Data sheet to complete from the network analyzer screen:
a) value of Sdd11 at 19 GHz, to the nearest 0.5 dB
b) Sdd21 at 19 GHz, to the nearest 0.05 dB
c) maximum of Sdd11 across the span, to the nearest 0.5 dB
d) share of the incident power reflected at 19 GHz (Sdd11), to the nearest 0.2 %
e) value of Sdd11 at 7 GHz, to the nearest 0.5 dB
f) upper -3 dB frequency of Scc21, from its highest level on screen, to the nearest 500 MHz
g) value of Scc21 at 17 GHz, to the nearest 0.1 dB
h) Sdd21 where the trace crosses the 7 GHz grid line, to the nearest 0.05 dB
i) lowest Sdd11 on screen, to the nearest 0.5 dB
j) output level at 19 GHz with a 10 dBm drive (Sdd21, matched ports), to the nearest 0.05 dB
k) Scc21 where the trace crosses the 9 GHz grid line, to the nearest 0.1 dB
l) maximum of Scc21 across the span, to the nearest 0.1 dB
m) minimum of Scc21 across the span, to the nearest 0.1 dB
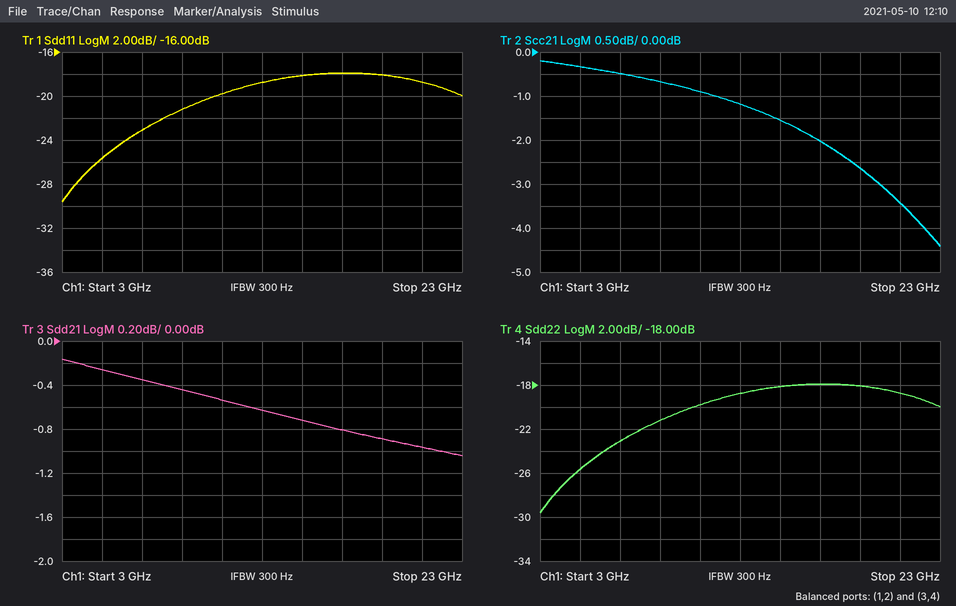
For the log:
-18.0 dB
-0.90 dB
-18.0 dB
1.6 %
-23.0 dB
20.5 GHz
-2.0 dB
-0.35 dB
-29.5 dB
9.10 dBm
-0.7 dB
-0.2 dB
-4.4 dB
